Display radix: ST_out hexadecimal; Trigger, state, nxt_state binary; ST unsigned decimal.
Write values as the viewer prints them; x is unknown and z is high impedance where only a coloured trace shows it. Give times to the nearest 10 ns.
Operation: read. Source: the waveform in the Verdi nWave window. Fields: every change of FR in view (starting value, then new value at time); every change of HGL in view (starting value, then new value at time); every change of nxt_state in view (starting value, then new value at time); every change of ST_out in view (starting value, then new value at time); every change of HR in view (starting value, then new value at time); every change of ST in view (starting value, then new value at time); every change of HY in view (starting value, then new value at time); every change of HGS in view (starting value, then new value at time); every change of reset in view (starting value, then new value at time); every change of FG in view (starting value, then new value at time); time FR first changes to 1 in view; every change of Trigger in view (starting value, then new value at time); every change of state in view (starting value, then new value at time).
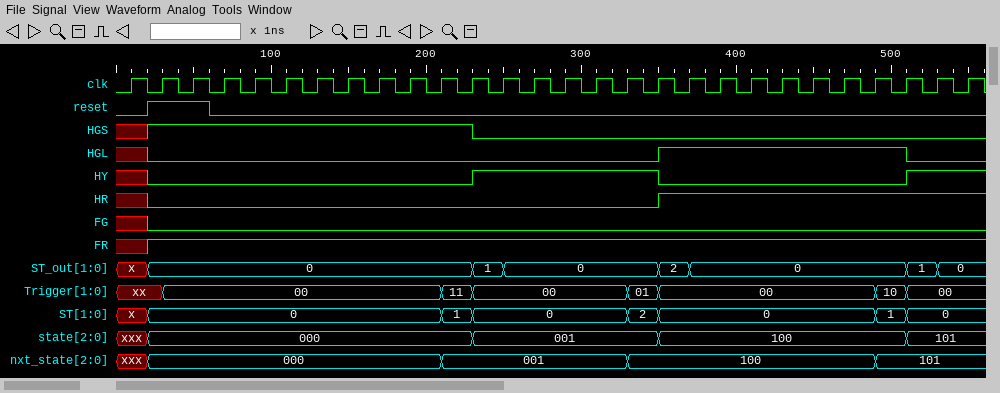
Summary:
x, 1 at 20 ns
x, 0 at 20 ns, 1 at 350 ns, 0 at 510 ns
xxx, 000 at 20 ns, 001 at 210 ns, 100 at 330 ns, 101 at 490 ns
x, 0 at 20 ns, 1 at 230 ns, 0 at 250 ns, 2 at 350 ns, 0 at 370 ns, 1 at 510 ns, 0 at 530 ns
x, 0 at 20 ns, 1 at 350 ns
x, 0 at 20 ns, 1 at 210 ns, 0 at 230 ns, 2 at 330 ns, 0 at 350 ns, 1 at 490 ns, 0 at 510 ns
x, 0 at 20 ns, 1 at 230 ns, 0 at 350 ns, 1 at 510 ns
x, 1 at 20 ns, 0 at 230 ns
0, 1 at 20 ns, 0 at 60 ns
x, 0 at 20 ns
20 ns
xx, 00 at 30 ns, 11 at 210 ns, 00 at 230 ns, 01 at 330 ns, 00 at 350 ns, 10 at 490 ns, 00 at 510 ns
xxx, 000 at 20 ns, 001 at 230 ns, 100 at 350 ns, 101 at 510 ns
